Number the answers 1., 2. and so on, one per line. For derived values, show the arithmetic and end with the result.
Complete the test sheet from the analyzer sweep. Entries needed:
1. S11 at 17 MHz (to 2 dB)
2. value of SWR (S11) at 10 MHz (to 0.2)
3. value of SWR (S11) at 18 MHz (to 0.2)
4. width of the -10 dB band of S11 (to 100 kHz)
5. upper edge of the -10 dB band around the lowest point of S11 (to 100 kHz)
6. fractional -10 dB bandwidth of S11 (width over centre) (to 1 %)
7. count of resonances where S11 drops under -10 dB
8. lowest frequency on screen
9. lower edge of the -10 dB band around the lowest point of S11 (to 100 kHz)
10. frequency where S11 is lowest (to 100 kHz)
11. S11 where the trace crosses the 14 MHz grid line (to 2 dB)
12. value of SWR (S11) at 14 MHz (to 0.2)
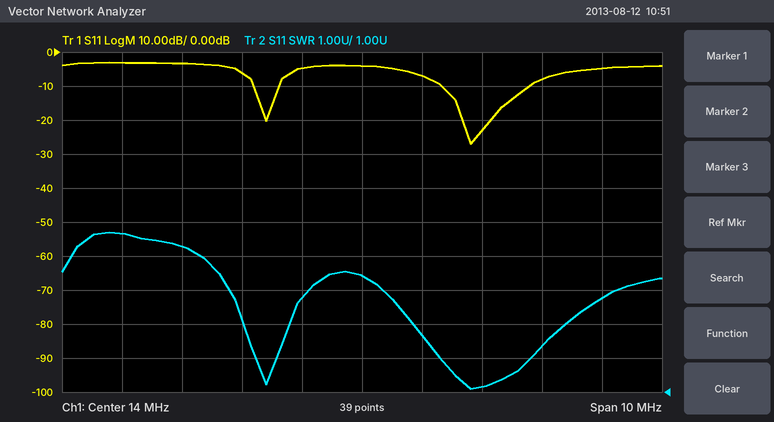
1. -8 dB
2. 5.6
3. 3.8
4. 16.8 MHz − 15.3 MHz = 1.5 MHz
5. 16.8 MHz
6. 1.5 MHz / 16.05 MHz ≈ 9 %
7. 2
8. 9 MHz
9. 15.3 MHz
10. 15.8 MHz
11. -4 dB
12. 4.4
